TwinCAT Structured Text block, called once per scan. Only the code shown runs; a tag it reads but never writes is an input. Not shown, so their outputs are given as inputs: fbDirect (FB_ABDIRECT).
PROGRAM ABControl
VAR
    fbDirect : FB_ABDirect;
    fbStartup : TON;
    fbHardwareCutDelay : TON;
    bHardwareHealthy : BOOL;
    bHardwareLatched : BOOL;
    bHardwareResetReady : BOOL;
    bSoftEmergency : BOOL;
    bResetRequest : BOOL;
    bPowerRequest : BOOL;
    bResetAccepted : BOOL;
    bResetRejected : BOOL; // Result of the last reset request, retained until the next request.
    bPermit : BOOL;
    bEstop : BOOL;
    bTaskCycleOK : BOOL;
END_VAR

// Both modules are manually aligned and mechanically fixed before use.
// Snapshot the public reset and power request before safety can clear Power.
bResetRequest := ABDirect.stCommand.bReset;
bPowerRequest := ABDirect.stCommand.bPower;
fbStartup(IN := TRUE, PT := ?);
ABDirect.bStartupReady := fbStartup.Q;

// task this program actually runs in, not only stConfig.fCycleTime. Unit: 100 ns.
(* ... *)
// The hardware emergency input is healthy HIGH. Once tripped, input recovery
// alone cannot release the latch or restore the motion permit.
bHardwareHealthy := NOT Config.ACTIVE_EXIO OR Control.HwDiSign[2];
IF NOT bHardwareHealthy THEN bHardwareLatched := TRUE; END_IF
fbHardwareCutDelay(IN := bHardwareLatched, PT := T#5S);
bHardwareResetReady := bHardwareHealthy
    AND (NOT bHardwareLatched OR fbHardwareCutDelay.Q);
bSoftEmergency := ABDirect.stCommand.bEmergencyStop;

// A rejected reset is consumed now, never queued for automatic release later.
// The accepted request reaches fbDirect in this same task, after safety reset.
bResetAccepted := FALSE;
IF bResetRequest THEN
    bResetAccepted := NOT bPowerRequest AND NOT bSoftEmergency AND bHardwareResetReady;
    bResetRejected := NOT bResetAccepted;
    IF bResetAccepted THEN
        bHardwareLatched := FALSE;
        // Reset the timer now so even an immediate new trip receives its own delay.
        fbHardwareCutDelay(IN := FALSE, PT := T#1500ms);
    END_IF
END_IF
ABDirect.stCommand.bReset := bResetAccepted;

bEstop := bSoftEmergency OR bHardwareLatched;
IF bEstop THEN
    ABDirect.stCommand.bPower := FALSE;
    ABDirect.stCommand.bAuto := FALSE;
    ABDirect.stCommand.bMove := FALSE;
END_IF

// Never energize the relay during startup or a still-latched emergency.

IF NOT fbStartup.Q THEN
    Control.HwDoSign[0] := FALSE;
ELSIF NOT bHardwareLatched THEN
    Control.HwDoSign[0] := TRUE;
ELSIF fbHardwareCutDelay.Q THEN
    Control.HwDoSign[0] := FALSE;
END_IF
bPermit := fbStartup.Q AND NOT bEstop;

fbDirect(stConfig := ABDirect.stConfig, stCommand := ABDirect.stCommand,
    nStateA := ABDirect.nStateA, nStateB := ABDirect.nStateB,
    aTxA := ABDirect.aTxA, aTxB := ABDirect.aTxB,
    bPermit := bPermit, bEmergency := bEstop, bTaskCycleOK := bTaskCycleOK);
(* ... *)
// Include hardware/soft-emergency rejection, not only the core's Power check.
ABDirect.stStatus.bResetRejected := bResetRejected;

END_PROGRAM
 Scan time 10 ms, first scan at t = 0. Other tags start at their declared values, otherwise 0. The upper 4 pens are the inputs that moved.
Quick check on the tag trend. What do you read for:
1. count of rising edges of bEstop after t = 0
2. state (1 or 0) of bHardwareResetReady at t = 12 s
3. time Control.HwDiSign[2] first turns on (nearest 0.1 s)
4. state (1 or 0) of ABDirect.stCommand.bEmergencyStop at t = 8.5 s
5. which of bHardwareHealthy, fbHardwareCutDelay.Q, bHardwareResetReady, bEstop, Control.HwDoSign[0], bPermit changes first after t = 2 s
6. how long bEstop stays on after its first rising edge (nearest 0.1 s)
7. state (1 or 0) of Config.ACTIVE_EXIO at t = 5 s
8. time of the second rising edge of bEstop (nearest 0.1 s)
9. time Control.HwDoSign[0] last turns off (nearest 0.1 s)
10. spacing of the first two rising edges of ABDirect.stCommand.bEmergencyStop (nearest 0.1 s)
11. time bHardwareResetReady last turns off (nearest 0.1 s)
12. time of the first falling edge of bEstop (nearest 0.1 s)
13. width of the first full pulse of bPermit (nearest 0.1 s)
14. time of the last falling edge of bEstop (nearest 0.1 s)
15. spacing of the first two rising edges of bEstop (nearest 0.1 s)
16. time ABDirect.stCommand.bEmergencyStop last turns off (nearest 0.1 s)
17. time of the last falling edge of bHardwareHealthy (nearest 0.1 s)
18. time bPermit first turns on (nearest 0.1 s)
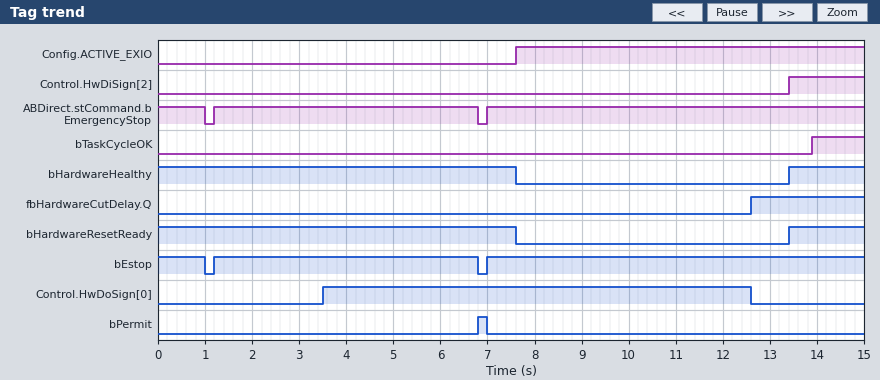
2
0
13.4 s
1
Control.HwDoSign[0]
5.6 s
0
7.0 s
12.6 s
5.8 s
7.6 s
1.0 s
0.2 s
6.8 s
5.8 s
6.8 s
7.6 s
6.8 s
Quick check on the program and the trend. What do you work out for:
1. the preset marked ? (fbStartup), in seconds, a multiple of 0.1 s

3.5 s
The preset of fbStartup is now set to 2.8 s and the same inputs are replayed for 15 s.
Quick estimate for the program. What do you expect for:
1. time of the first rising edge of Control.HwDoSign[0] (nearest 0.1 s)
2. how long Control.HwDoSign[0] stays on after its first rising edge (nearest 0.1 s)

2.8 s
9.8 s
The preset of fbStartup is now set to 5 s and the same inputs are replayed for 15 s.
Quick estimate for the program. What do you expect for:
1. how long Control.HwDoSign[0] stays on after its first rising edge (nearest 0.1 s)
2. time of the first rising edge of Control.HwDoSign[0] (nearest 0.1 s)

7.6 s
5.0 s
